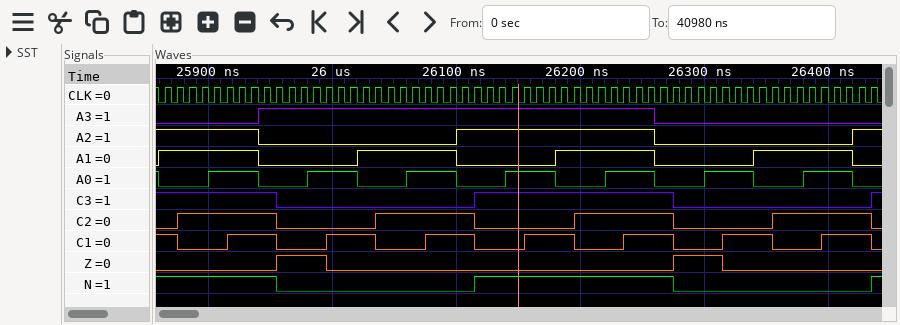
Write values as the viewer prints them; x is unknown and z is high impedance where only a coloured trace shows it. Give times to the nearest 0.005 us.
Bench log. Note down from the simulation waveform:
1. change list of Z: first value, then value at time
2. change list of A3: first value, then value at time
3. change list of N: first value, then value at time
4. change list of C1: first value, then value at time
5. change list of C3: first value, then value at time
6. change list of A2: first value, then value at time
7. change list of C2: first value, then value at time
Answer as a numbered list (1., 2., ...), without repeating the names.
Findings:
1. 0, 1 at 25.955 us, 0 at 25.995 us, 1 at 26.275 us, 0 at 26.315 us
2. 0, 1 at 25.94 us, 0 at 26.26 us
3. 1, 0 at 25.955 us, 1 at 26.115 us, 0 at 26.275 us, 1 at 26.435 us
4. 1, 0 at 25.875 us, 1 at 25.915 us, 0 at 25.955 us, 1 at 25.995 us, 0 at 26.035 us, 1 at 26.075 us, 0 at 26.115 us, 1 at 26.155 us, 0 at 26.195 us, 1 at 26.235 us, 0 at 26.275 us, 1 at 26.315 us, 0 at 26.355 us, 1 at 26.395 us, 0 at 26.435 us
5. 1, 0 at 25.955 us, 1 at 26.115 us, 0 at 26.275 us, 1 at 26.435 us
6. 1, 0 at 25.94 us, 1 at 26.1 us, 0 at 26.26 us, 1 at 26.42 us
7. 0, 1 at 25.875 us, 0 at 25.955 us, 1 at 26.035 us, 0 at 26.115 us, 1 at 26.195 us, 0 at 26.275 us, 1 at 26.355 us, 0 at 26.435 us
